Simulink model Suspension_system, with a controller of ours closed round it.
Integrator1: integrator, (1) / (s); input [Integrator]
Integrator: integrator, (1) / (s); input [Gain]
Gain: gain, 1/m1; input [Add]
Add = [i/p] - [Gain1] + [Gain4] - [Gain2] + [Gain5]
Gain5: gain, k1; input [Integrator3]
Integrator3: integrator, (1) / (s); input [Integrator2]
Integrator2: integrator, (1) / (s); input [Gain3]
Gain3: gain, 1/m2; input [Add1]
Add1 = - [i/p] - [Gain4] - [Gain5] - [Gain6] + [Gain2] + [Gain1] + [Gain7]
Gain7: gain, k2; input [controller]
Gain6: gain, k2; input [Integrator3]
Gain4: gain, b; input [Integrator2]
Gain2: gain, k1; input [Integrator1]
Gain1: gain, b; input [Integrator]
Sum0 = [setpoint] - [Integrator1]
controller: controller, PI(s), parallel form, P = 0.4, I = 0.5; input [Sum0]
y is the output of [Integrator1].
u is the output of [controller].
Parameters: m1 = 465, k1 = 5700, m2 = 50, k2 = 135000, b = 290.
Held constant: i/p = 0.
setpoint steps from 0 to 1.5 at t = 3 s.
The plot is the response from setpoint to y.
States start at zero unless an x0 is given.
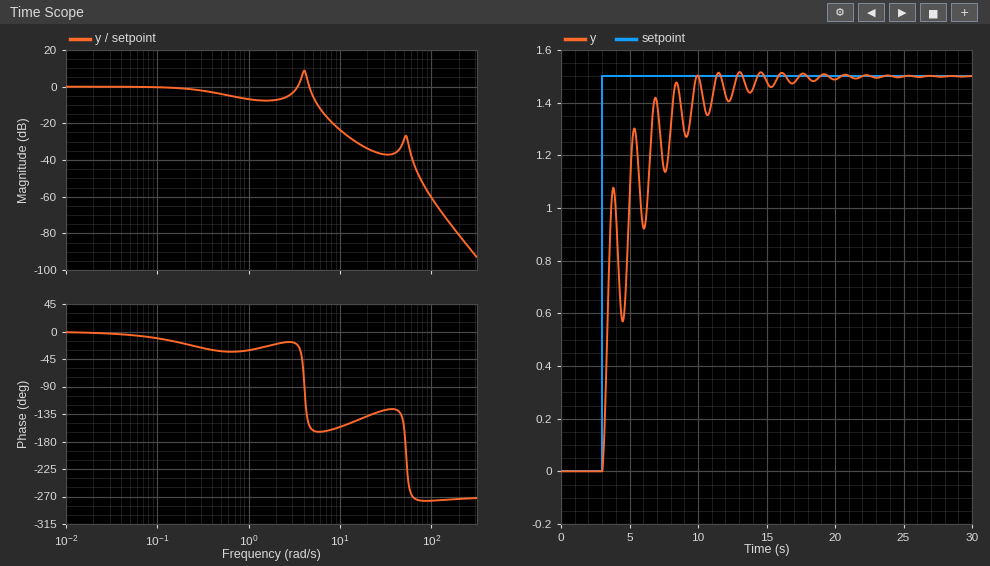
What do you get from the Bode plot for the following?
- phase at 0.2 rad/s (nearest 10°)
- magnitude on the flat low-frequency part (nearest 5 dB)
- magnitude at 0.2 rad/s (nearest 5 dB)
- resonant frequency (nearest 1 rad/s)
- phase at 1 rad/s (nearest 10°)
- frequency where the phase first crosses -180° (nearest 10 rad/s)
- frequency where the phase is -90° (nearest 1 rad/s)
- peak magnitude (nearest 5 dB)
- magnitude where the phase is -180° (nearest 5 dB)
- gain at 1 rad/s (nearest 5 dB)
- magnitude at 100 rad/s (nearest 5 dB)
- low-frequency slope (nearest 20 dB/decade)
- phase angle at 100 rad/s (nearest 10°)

-20°
0 dB
0 dB
4 rad/s
-30°
50 rad/s
4 rad/s
10 dB
-25 dB
-5 dB
-60 dB
0 dB/decade
-280°
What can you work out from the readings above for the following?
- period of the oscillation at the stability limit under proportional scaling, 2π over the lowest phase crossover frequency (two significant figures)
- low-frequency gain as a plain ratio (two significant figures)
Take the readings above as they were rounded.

0.13 s
1.0
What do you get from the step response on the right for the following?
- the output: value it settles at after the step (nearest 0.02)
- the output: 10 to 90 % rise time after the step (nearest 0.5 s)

1.50
3.5 s
